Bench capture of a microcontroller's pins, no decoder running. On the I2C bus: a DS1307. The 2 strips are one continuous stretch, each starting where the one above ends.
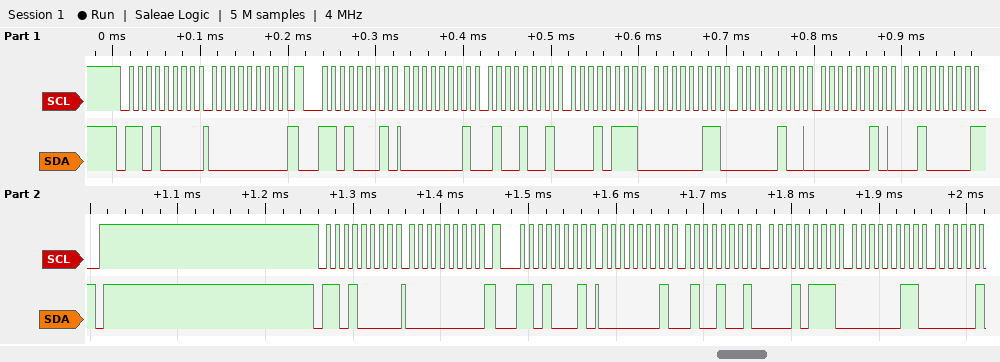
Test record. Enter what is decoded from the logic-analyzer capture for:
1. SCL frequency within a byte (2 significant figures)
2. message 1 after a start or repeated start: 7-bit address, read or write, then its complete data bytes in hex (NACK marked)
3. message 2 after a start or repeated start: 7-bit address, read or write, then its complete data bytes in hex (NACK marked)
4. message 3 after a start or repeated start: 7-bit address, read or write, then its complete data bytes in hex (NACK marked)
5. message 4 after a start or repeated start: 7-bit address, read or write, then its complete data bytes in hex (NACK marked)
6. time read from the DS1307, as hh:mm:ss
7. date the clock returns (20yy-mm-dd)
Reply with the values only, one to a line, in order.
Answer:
100 kHz
0x68 write: 00
0x68 read: 01 49 17 03 04 02 20 NACK
0x68 write: 00
0x68 read: 01 49 17 03
17:49:01
2020-02-04
